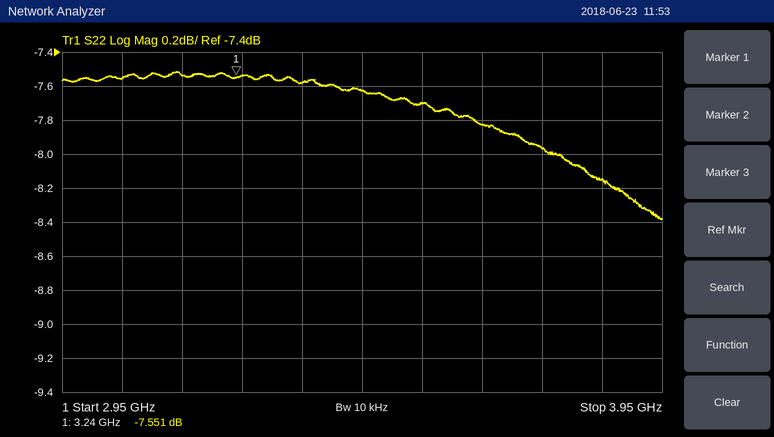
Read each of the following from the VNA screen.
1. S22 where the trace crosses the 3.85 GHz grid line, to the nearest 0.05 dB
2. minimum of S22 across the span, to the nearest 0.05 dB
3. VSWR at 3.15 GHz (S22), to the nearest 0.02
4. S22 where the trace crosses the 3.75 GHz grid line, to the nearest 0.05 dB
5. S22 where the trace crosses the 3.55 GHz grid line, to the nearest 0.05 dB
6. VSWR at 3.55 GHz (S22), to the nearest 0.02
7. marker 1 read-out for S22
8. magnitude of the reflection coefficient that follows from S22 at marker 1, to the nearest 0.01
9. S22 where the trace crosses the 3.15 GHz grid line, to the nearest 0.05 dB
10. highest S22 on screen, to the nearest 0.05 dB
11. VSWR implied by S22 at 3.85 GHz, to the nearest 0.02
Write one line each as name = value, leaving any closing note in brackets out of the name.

S22 where the trace crosses the 3.85 GHz grid line, to the nearest 0.05 dB = -8.15 dB
minimum of S22 across the span, to the nearest 0.05 dB = -8.40 dB
VSWR at 3.15 GHz (S22), to the nearest 0.02 = 2.44
S22 where the trace crosses the 3.75 GHz grid line, to the nearest 0.05 dB = -7.95 dB
S22 where the trace crosses the 3.55 GHz grid line, to the nearest 0.05 dB = -7.70 dB
VSWR at 3.55 GHz (S22), to the nearest 0.02 = 2.40
marker 1 read-out for S22 = -7.551 dB
magnitude of the reflection coefficient that follows from S22 at marker 1, to the nearest 0.01 = 0.42
S22 where the trace crosses the 3.15 GHz grid line, to the nearest 0.05 dB = -7.55 dB
highest S22 on screen, to the nearest 0.05 dB = -7.50 dB
VSWR implied by S22 at 3.85 GHz, to the nearest 0.02 = 2.28
